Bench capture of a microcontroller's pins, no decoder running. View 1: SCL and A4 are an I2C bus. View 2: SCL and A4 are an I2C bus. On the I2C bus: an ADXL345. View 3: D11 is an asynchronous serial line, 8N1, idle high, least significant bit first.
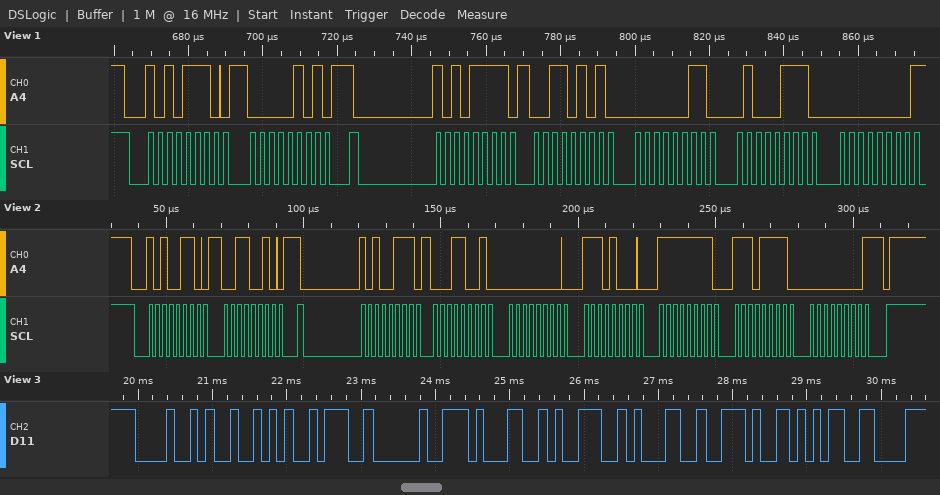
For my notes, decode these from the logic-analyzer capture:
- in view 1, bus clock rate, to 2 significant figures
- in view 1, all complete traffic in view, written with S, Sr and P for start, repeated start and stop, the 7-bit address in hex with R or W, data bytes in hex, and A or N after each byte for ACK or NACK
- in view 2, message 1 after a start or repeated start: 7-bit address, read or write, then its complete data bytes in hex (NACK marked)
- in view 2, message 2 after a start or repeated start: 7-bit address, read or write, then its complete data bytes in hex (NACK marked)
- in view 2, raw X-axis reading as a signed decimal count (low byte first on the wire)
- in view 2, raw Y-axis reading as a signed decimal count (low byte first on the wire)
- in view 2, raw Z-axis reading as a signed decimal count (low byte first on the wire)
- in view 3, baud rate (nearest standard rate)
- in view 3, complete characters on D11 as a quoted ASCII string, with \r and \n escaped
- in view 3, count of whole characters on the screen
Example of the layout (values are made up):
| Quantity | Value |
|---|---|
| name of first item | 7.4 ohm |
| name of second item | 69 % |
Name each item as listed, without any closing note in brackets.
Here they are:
| Quantity | Value |
|---|---|
| in view 1, bus clock rate, to 2 significant figures | 400 kHz |
| in view 1, all complete traffic in view, written with S, Sr and P for start, repeated start and stop, the 7-bit address in hex with R or W, data bytes in hex, and A or N after each byte for ACK or NACK | S 57W A 05 A Sr 57R A 35 A 03 A 47 A 00 N |
| in view 2, message 1 after a start or repeated start: 7-bit address, read or write, then its complete data bytes in hex | 0x53 write: 32 |
| in view 2, message 2 after a start or repeated start: 7-bit address, read or write, then its complete data bytes in hex | 0x53 read: 19 00 E8 FF EF 00 NACK |
| in view 2, raw X-axis reading as a signed decimal count | 25 |
| in view 2, raw Y-axis reading as a signed decimal count | -24 |
| in view 2, raw Z-axis reading as a signed decimal count | 239 |
| in view 3, baud rate | 9600 baud |
| in view 3, complete characters on D11 as a quoted ASCII string, with \r and \n escaped | "HR: 191.5" |
| in view 3, count of whole characters on the screen | 9 |
